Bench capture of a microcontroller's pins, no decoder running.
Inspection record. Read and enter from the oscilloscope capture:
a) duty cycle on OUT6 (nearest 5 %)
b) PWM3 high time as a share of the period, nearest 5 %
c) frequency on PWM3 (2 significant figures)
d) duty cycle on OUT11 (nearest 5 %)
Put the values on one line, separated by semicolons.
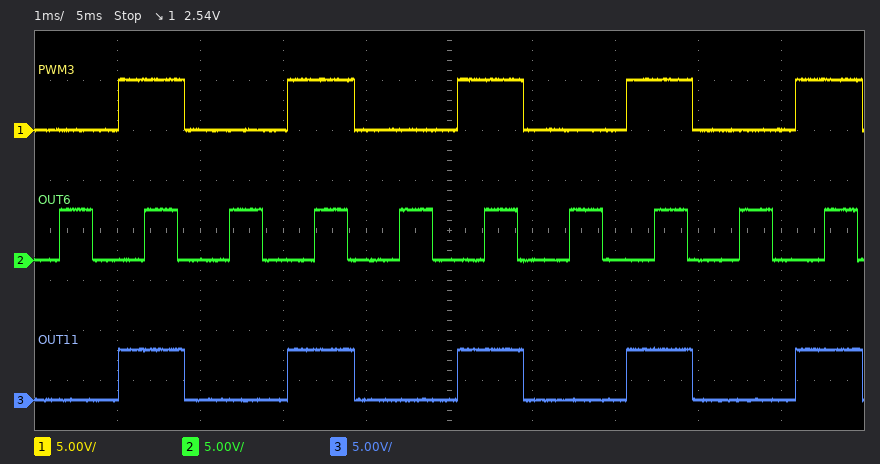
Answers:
40 %; 40 %; 490 Hz; 40 %
